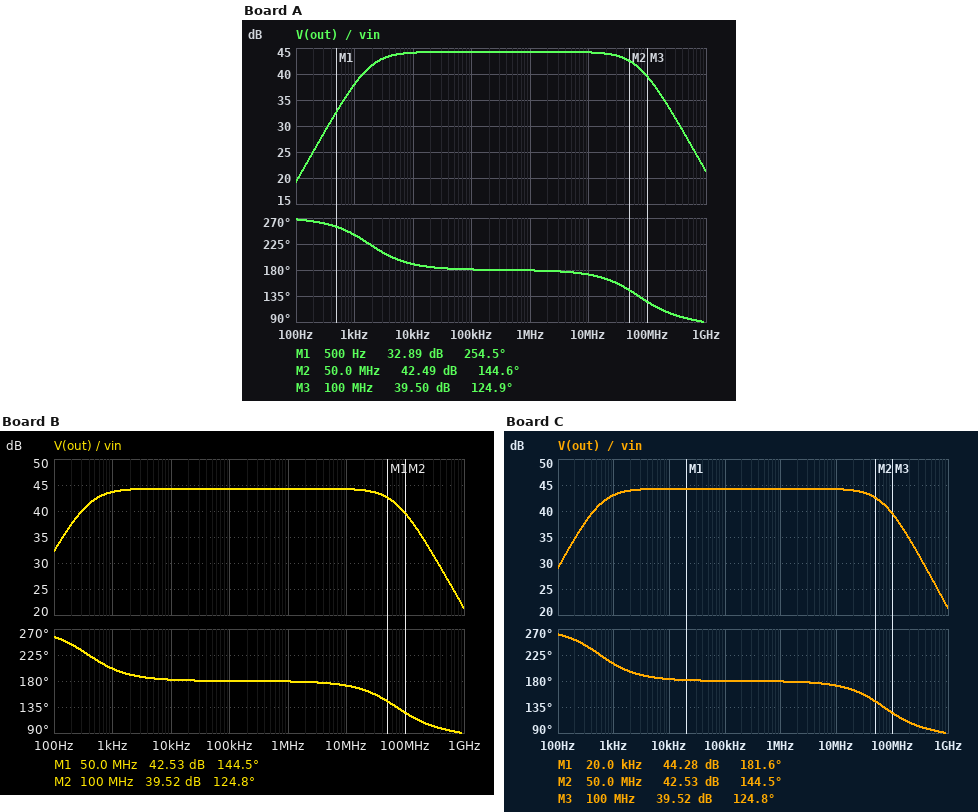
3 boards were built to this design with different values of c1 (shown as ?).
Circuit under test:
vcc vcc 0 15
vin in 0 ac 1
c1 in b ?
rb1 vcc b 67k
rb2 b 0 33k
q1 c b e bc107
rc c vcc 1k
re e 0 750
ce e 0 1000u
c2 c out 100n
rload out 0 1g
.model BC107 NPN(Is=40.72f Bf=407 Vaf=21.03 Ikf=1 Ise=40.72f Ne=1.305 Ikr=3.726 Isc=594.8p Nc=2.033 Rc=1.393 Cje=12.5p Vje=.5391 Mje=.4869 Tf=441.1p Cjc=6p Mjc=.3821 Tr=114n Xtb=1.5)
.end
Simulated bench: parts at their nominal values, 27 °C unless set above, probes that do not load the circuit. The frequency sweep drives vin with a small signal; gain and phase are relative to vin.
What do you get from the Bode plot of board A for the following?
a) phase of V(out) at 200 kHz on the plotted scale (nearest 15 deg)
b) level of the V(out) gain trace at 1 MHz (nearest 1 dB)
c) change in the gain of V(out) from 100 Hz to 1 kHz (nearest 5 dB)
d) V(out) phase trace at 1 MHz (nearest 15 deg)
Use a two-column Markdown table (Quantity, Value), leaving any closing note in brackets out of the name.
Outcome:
| Quantity | Value |
|---|---|
| phase of V(out) at 200 kHz on the plotted scale | 180 deg |
| level of the V(out) gain trace at 1 MHz | 44 dB |
| change in the gain of V(out) from 100 Hz to 1 kHz | 20 dB |
| V(out) phase trace at 1 MHz | 180 deg |
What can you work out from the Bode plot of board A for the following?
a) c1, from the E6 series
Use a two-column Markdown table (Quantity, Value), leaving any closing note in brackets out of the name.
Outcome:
| Quantity | Value |
|---|---|
| c1, from the E6 series | 68 nF |
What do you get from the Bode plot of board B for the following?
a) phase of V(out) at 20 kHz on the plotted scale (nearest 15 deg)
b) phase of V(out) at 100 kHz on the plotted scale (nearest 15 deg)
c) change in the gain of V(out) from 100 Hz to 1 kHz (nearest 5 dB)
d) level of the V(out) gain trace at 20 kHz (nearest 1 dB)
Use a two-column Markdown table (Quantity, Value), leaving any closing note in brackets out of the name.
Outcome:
| Quantity | Value |
|---|---|
| phase of V(out) at 20 kHz on the plotted scale | 180 deg |
| phase of V(out) at 100 kHz on the plotted scale | 180 deg |
| change in the gain of V(out) from 100 Hz to 1 kHz | 10 dB |
| level of the V(out) gain trace at 20 kHz | 44 dB |
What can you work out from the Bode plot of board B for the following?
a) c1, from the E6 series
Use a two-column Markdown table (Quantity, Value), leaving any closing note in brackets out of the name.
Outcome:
| Quantity | Value |
|---|---|
| c1, from the E6 series | 330 nF |
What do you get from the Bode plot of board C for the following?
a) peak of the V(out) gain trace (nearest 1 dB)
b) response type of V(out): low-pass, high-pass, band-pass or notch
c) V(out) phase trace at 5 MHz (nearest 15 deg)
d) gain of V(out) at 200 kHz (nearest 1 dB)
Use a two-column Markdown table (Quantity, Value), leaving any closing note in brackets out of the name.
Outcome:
| Quantity | Value |
|---|---|
| peak of the V(out) gain trace | 44 dB |
| response type of V(out): low-pass, high-pass, band-pass or notch | band-pass |
| V(out) phase trace at 5 MHz | 180 deg |
| gain of V(out) at 200 kHz | 44 dB |
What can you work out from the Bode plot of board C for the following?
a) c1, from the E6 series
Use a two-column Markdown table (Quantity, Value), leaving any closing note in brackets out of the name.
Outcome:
| Quantity | Value |
|---|---|
| c1, from the E6 series | 220 nF |
